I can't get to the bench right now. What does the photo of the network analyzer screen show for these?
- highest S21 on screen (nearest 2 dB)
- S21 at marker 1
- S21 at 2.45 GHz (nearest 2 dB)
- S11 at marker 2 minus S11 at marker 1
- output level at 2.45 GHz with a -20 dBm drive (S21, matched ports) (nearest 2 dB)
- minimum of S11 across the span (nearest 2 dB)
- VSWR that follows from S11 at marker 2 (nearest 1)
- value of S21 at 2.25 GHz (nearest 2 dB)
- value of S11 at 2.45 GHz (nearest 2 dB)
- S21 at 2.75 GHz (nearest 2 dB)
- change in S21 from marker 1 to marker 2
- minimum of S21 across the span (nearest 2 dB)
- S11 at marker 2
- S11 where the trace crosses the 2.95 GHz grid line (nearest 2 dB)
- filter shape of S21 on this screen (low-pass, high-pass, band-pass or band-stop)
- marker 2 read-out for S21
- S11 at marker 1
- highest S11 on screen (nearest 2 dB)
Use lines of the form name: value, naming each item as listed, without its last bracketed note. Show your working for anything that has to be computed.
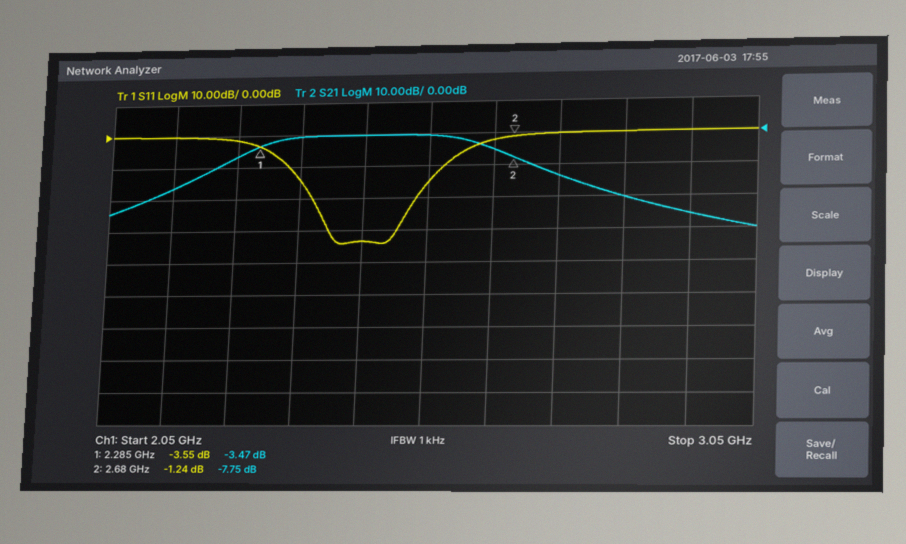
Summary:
highest S21 on screen: 0 dB
S21 at marker 1: -3.47 dB
S21 at 2.45 GHz: 0 dB
S11 at marker 2 minus S11 at marker 1: -1.24 − (-3.55) = 2.31 dB
output level at 2.45 GHz with a -20 dBm drive (S21, matched ports): -20 dBm + (0 dB) = -20 dBm
minimum of S11 across the span: -34 dB
VSWR that follows from S11 at marker 2: (1 + 0.8670)/(1 − 0.8670) ≈ 14
value of S21 at 2.25 GHz: -6 dB
value of S11 at 2.45 GHz: -34 dB
S21 at 2.75 GHz: -14 dB
change in S21 from marker 1 to marker 2: -7.75 − (-3.47) = -4.28 dB
minimum of S21 across the span: -30 dB
S11 at marker 2: -1.24 dB
S11 where the trace crosses the 2.95 GHz grid line: 0 dB
filter shape of S21 on this screen: band-pass
marker 2 read-out for S21: -7.75 dB
S11 at marker 1: -3.55 dB
highest S11 on screen: 0 dB
